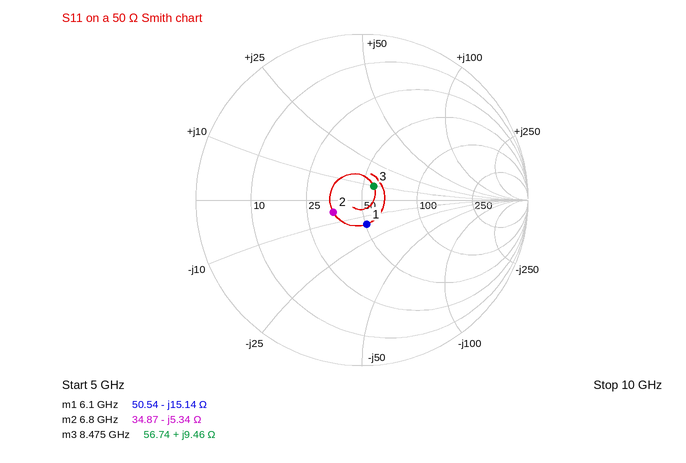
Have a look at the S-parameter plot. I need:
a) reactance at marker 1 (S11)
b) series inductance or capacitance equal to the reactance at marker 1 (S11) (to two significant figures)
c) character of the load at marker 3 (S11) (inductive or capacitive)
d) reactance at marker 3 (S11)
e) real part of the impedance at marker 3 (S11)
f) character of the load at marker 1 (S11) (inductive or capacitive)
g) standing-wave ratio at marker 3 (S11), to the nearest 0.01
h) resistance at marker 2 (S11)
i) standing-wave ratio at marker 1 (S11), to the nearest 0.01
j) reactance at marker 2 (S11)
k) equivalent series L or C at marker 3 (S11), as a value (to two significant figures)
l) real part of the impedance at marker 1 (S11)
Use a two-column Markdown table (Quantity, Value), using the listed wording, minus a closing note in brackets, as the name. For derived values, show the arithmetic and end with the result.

| Quantity | Value |
|---|---|
| reactance at marker 1 | -15.14 Ω |
| series inductance or capacitance equal to the reactance at marker 1 (S11) | C = 1/(2π × 6.1 GHz × 15.14 Ω) ≈ 1.7 pF |
| character of the load at marker 3 (S11) | inductive |
| reactance at marker 3 | +9.46 Ω |
| real part of the impedance at marker 3 | 56.74 Ω |
| character of the load at marker 1 (S11) | capacitive |
| standing-wave ratio at marker 3 (S11), to the nearest 0.01 | 1.24 |
| resistance at marker 2 | 34.87 Ω |
| standing-wave ratio at marker 1 (S11), to the nearest 0.01 | 1.35 |
| reactance at marker 2 | -5.34 Ω |
| equivalent series L or C at marker 3 (S11), as a value | L = 9.46 Ω/(2π × 8.475 GHz) ≈ 178 pH, so 180 pH to two significant figures |
| real part of the impedance at marker 1 | 50.54 Ω |
